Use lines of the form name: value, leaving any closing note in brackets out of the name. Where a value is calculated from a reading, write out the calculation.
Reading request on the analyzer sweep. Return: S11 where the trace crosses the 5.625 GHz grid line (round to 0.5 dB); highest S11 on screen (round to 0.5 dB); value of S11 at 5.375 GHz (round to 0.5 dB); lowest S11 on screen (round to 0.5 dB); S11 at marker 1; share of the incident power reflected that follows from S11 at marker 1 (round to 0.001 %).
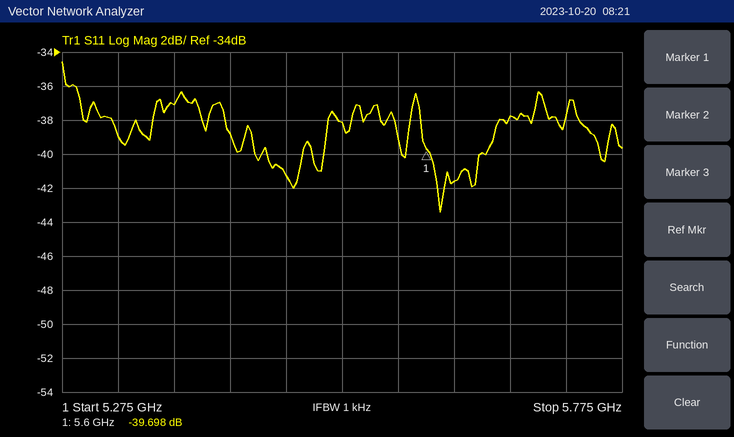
S11 where the trace crosses the 5.625 GHz grid line: -41.5 dB
highest S11 on screen: -34.5 dB
value of S11 at 5.375 GHz: -37.0 dB
lowest S11 on screen: -43.5 dB
S11 at marker 1: -39.698 dB
share of the incident power reflected that follows from S11 at marker 1: 10^(-39.698/10) ≈ 0.011 %
